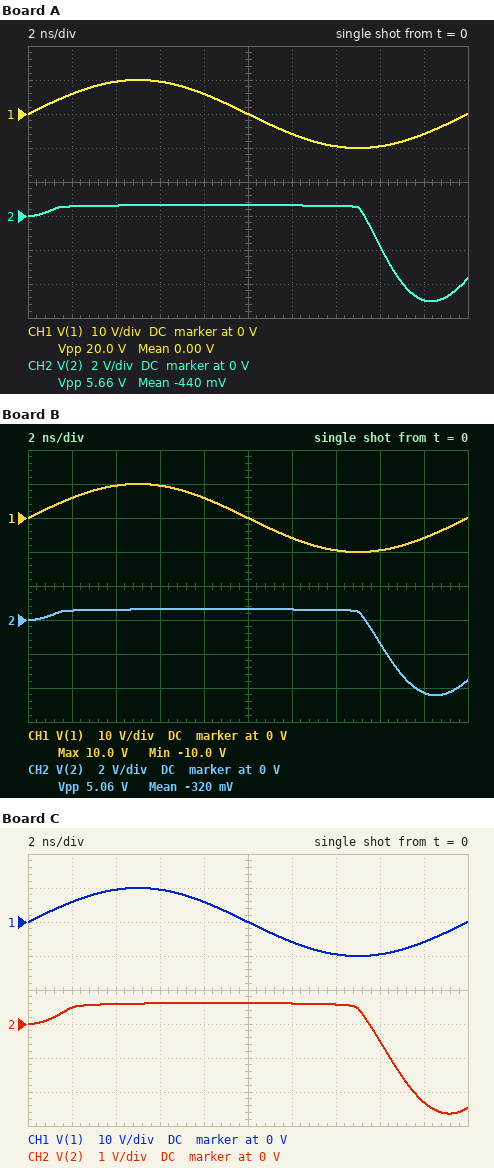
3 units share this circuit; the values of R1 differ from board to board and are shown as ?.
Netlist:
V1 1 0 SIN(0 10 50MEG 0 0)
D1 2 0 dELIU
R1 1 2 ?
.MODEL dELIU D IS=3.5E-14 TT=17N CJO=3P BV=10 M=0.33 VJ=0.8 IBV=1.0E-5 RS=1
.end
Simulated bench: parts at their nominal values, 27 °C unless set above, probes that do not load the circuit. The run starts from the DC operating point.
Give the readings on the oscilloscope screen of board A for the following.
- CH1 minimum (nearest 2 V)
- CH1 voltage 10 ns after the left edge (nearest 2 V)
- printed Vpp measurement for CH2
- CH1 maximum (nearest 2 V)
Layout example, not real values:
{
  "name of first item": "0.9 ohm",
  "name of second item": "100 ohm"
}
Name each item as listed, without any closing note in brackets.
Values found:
{
  "CH1 minimum": "-10 V",
  "CH1 voltage 10 ns after the left edge": "0 V",
  "printed Vpp measurement for CH2": "5.66 V",
  "CH1 maximum": "10 V"
}
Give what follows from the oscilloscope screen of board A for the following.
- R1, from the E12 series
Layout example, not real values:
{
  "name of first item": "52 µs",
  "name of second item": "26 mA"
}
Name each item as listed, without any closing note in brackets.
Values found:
{
  "R1, from the E12 series": "1.5 kΩ"
}
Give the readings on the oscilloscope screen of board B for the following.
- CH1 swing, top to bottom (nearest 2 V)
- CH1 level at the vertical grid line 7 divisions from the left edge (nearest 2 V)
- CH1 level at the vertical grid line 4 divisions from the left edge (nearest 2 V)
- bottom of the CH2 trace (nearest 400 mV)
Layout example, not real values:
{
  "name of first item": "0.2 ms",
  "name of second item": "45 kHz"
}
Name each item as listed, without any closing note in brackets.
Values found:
{
  "CH1 swing, top to bottom": "20 V",
  "CH1 level at the vertical grid line 7 divisions from the left edge": "-10 V",
  "CH1 level at the vertical grid line 4 divisions from the left edge": "6 V",
  "bottom of the CH2 trace": "-4.4 V"
}
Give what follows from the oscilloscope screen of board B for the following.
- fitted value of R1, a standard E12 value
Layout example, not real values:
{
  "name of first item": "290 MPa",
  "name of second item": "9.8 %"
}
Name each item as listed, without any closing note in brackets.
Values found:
{
  "fitted value of R1, a standard E12 value": "1.8 kΩ"
}
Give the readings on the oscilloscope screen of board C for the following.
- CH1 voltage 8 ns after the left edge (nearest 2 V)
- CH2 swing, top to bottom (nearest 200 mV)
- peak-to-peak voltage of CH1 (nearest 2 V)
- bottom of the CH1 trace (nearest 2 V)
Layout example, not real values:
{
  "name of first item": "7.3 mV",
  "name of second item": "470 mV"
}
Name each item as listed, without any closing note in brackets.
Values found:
{
  "CH1 voltage 8 ns after the left edge": "6 V",
  "CH2 swing, top to bottom": "3.2 V",
  "peak-to-peak voltage of CH1": "20 V",
  "bottom of the CH1 trace": "-10 V"
}
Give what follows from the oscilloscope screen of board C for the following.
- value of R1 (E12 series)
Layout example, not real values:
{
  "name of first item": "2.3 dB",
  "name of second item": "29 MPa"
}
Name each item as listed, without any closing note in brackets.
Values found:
{
  "value of R1": "3.3 kΩ"
}
